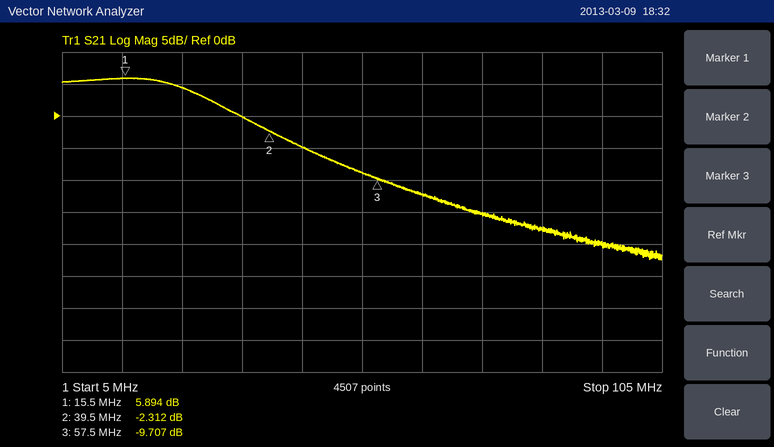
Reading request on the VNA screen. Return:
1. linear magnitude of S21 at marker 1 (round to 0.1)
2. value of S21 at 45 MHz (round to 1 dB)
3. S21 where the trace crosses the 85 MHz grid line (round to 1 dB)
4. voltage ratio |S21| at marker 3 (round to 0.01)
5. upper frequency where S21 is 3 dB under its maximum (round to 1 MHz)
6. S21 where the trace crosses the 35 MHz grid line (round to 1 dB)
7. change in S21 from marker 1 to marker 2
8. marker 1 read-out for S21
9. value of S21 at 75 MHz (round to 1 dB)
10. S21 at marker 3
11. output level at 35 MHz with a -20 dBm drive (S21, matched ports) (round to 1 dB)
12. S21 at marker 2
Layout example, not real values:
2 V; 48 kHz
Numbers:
2.0; -5 dB; -18 dB; 0.33; 29 MHz; 0 dB; -8.206 dB; 5.894 dB; -15 dB; -9.707 dB; -20 dBm; -2.312 dB
